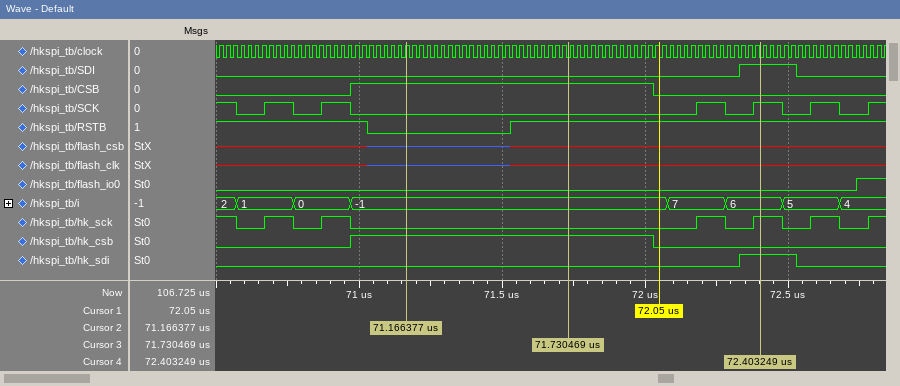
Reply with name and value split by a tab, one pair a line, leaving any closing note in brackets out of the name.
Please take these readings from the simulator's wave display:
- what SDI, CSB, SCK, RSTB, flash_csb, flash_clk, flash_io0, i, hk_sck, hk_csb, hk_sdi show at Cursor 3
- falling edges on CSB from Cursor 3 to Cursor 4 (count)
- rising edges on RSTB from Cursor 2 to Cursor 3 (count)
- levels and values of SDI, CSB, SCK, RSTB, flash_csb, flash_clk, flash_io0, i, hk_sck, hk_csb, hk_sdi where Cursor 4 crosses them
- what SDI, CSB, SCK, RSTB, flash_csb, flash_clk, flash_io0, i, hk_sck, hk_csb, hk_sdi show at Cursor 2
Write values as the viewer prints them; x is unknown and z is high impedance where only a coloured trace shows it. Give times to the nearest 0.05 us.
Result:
what SDI, CSB, SCK, RSTB, flash_csb, flash_clk, flash_io0, i, hk_sck, hk_csb, hk_sdi show at Cursor 3	SDI=0, CSB=1, SCK=0, RSTB=1, flash_csb=x, flash_clk=x, flash_io0=0, i=-1, hk_sck=0, hk_csb=1, hk_sdi=0
falling edges on CSB from Cursor 3 to Cursor 4	1
rising edges on RSTB from Cursor 2 to Cursor 3	1
levels and values of SDI, CSB, SCK, RSTB, flash_csb, flash_clk, flash_io0, i, hk_sck, hk_csb, hk_sdi where Cursor 4 crosses them	SDI=1, CSB=0, SCK=1, RSTB=1, flash_csb=x, flash_clk=x, flash_io0=0, i=6, hk_sck=1, hk_csb=0, hk_sdi=1
what SDI, CSB, SCK, RSTB, flash_csb, flash_clk, flash_io0, i, hk_sck, hk_csb, hk_sdi show at Cursor 2	SDI=0, CSB=1, SCK=0, RSTB=0, flash_csb=z, flash_clk=z, flash_io0=0, i=-1, hk_sck=0, hk_csb=1, hk_sdi=0
